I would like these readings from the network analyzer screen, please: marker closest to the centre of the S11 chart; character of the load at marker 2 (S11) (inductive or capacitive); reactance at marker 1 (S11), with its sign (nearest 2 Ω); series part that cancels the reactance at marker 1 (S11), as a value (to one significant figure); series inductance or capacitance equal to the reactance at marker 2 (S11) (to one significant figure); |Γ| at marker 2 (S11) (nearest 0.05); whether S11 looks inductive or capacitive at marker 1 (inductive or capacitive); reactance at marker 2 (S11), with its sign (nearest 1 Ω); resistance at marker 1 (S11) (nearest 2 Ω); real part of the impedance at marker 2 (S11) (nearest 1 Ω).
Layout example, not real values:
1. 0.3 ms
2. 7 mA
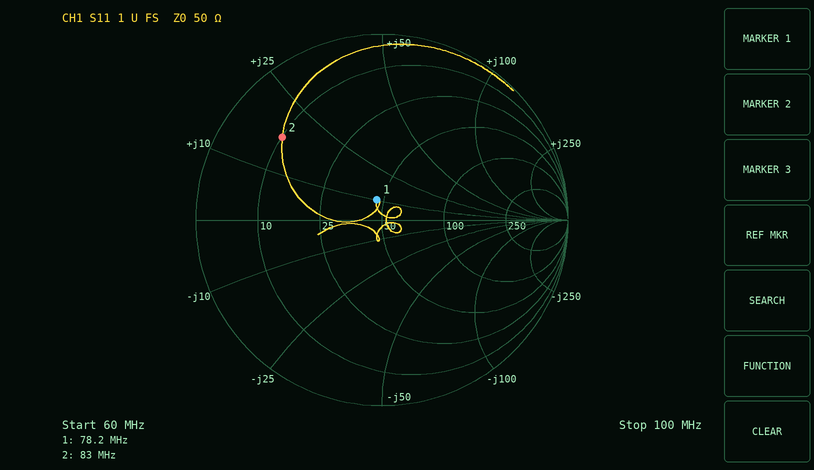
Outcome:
1. marker 1
2. inductive
3. +10 Ω
4. 200 pF
5. 30 nH
6. 0.70
7. inductive
8. +17 Ω
9. 46 Ω
10. 10 Ω
